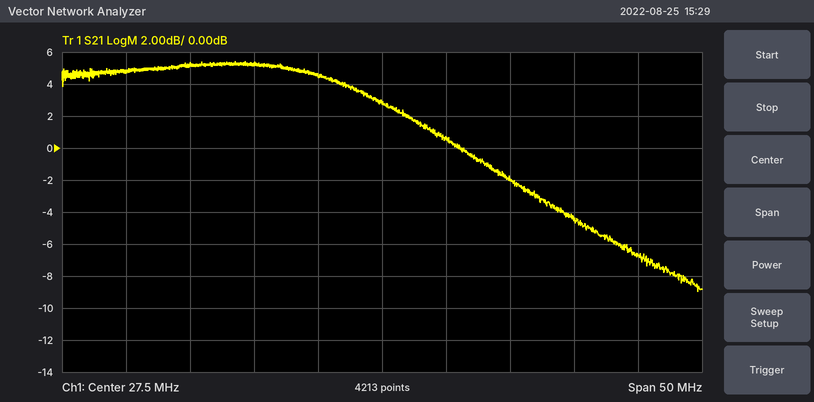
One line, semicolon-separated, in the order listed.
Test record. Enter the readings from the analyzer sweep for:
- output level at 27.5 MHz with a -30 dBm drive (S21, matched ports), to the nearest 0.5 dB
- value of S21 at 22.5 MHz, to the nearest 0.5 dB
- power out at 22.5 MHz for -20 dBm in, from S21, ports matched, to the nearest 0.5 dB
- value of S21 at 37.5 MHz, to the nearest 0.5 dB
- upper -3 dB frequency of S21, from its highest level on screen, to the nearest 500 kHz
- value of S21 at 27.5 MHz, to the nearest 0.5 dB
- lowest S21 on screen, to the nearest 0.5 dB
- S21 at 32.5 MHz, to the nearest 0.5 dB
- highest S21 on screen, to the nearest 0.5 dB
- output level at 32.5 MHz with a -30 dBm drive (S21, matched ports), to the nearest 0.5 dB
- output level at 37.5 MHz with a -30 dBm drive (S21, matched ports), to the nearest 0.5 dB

-27.0 dBm; 4.5 dB; -15.5 dBm; -2.0 dB; 28.5 MHz; 3.0 dB; -9.0 dB; 0.5 dB; 5.5 dB; -29.5 dBm; -32.0 dBm
